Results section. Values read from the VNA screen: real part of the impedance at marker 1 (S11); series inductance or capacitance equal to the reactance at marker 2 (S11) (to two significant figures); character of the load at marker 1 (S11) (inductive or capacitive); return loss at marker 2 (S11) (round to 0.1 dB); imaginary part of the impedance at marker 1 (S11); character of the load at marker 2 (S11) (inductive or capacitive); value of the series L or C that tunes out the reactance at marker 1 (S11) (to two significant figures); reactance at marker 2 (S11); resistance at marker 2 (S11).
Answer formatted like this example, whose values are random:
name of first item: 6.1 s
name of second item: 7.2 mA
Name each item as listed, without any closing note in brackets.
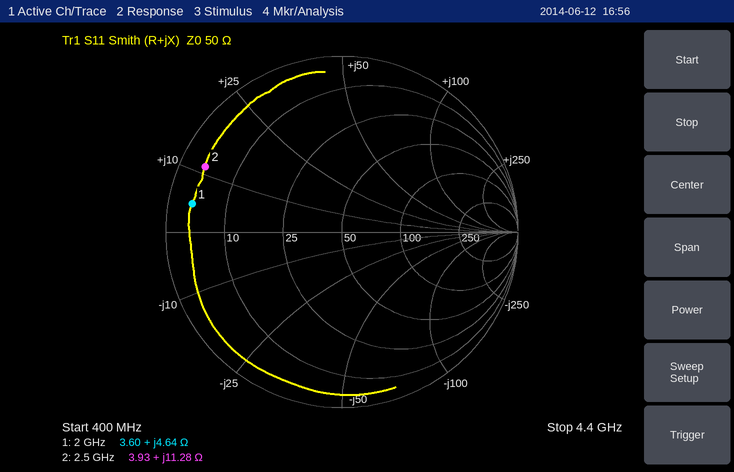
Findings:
real part of the impedance at marker 1: 3.60 Ω
series inductance or capacitance equal to the reactance at marker 2 (S11): 720 pH
character of the load at marker 1 (S11): inductive
return loss at marker 2 (S11): 1.3 dB
imaginary part of the impedance at marker 1: +4.64 Ω
character of the load at marker 2 (S11): inductive
value of the series L or C that tunes out the reactance at marker 1 (S11): 17 pF
reactance at marker 2: +11.28 Ω
resistance at marker 2: 3.93 Ω
